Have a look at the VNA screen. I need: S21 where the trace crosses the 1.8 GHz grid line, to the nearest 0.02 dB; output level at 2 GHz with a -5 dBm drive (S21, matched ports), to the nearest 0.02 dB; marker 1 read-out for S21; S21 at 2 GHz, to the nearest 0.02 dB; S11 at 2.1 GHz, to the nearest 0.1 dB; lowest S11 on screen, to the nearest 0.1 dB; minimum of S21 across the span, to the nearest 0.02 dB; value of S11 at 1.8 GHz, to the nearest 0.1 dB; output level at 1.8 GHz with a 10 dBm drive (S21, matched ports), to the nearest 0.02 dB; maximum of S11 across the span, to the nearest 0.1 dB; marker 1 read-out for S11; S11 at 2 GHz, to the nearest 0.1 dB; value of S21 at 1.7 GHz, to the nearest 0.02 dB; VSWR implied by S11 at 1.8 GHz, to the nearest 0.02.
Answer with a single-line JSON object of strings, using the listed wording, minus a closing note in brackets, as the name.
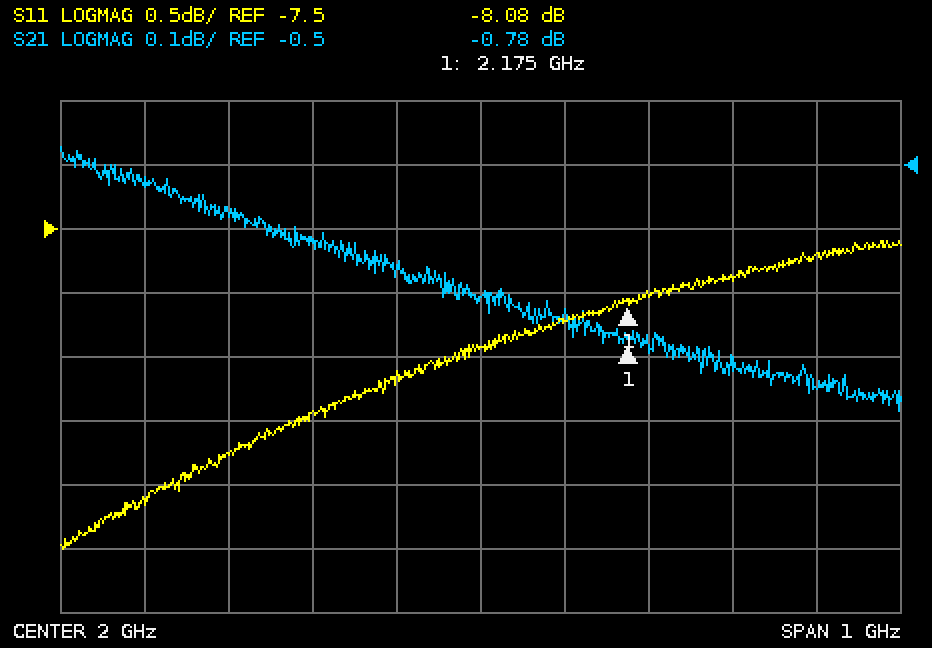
{"S21 where the trace crosses the 1.8 GHz grid line, to the nearest 0.02 dB": "-0.62 dB", "output level at 2 GHz with a -5 dBm drive (S21, matched ports), to the nearest 0.02 dB": "-5.70 dBm", "marker 1 read-out for S21": "-0.78 dB", "S21 at 2 GHz, to the nearest 0.02 dB": "-0.70 dB", "S11 at 2.1 GHz, to the nearest 0.1 dB": "-8.2 dB", "lowest S11 on screen, to the nearest 0.1 dB": "-10.0 dB", "minimum of S21 across the span, to the nearest 0.02 dB": "-0.88 dB", "value of S11 at 1.8 GHz, to the nearest 0.1 dB": "-8.9 dB", "output level at 1.8 GHz with a 10 dBm drive (S21, matched ports), to the nearest 0.02 dB": "9.38 dBm", "maximum of S11 across the span, to the nearest 0.1 dB": "-7.6 dB", "marker 1 read-out for S11": "-8.08 dB", "S11 at 2 GHz, to the nearest 0.1 dB": "-8.4 dB", "value of S21 at 1.7 GHz, to the nearest 0.02 dB": "-0.58 dB", "VSWR implied by S11 at 1.8 GHz, to the nearest 0.02": "2.12"}
